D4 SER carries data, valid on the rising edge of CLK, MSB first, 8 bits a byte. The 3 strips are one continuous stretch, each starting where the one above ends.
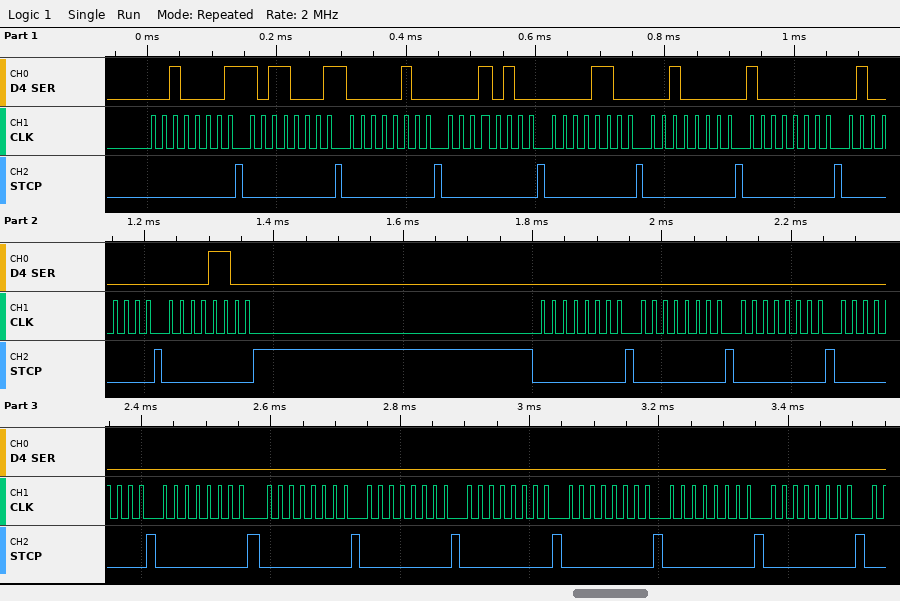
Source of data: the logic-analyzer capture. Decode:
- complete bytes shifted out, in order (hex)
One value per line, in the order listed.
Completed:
21 B1 04 14 0C 20 80 40 0C 00 00 00 00 00 00 00 00 00 00 00
